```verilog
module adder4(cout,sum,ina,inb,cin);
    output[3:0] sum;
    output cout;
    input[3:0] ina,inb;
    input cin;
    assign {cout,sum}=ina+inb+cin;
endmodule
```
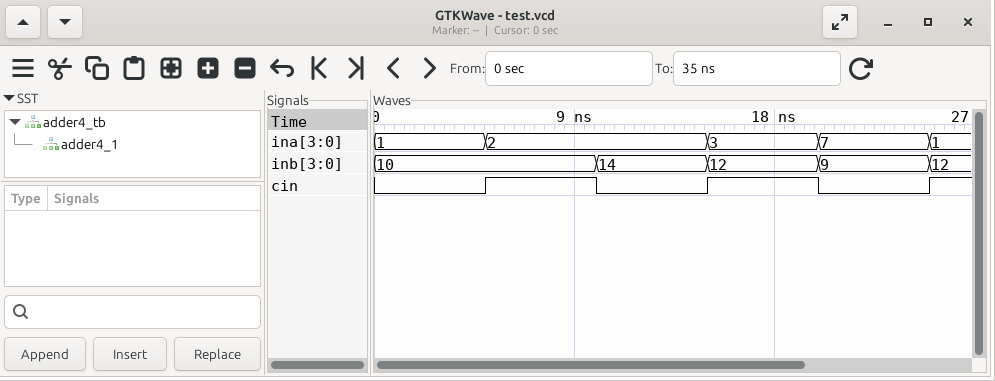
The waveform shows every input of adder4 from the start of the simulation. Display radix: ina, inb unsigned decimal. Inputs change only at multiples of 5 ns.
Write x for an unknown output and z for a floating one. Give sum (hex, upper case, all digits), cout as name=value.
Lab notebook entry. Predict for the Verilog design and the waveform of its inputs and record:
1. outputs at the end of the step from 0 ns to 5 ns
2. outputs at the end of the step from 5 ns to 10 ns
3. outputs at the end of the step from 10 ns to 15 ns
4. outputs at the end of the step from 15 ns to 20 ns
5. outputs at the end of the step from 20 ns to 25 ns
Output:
sum=B, cout=0
sum=D, cout=0
sum=0, cout=1
sum=0, cout=1
sum=0, cout=1
